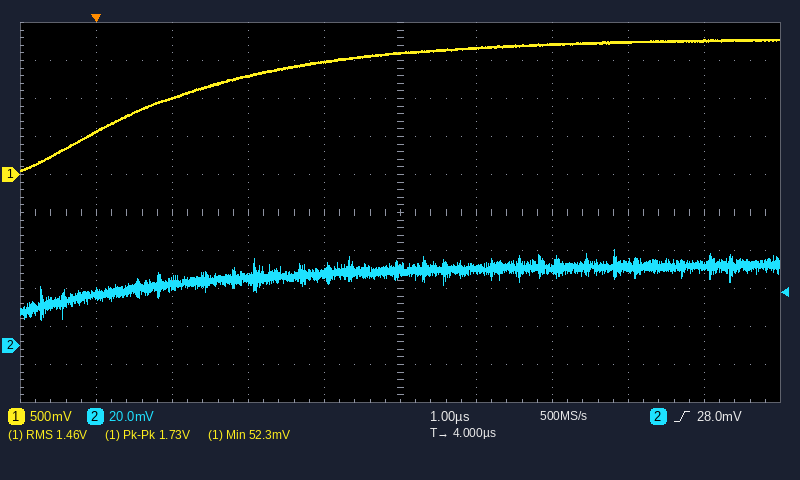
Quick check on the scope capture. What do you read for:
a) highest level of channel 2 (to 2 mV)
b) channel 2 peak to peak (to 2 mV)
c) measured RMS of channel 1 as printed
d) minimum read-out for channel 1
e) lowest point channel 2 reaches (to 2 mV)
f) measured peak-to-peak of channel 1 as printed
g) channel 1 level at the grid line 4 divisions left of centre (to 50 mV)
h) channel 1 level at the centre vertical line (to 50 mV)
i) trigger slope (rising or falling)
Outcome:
50 mV
36 mV
1.46 V
52.3 mV
14 mV
1.73 V
550 mV
1.60 V
rising
